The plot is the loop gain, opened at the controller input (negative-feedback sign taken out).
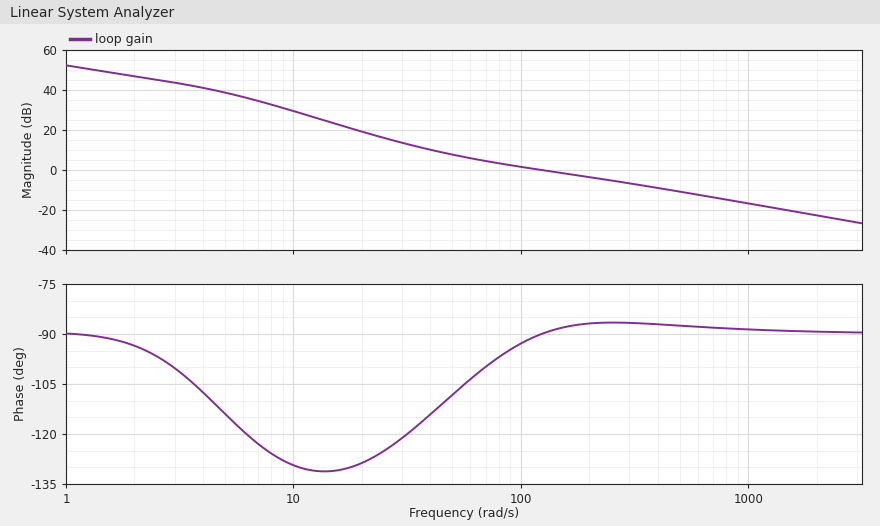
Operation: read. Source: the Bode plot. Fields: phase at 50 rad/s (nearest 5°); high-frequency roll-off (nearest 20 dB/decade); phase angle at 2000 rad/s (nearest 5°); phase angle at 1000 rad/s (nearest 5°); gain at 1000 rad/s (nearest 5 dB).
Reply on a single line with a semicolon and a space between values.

-110°; -20 dB/decade; -90°; -90°; -15 dB
